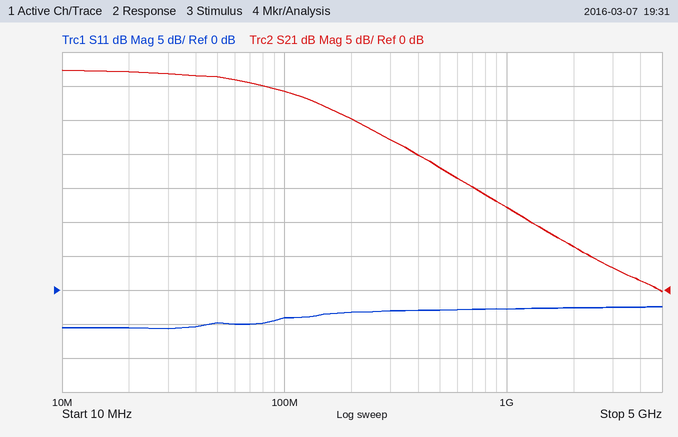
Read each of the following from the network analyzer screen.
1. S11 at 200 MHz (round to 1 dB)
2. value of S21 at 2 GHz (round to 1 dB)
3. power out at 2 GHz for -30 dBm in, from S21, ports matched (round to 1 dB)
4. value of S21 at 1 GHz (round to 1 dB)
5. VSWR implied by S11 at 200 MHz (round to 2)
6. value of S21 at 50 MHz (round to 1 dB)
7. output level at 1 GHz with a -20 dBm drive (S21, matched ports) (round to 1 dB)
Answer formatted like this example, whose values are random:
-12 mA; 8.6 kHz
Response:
-3 dB; 6 dB; -24 dBm; 12 dB; 6; 31 dB; -8 dBm
